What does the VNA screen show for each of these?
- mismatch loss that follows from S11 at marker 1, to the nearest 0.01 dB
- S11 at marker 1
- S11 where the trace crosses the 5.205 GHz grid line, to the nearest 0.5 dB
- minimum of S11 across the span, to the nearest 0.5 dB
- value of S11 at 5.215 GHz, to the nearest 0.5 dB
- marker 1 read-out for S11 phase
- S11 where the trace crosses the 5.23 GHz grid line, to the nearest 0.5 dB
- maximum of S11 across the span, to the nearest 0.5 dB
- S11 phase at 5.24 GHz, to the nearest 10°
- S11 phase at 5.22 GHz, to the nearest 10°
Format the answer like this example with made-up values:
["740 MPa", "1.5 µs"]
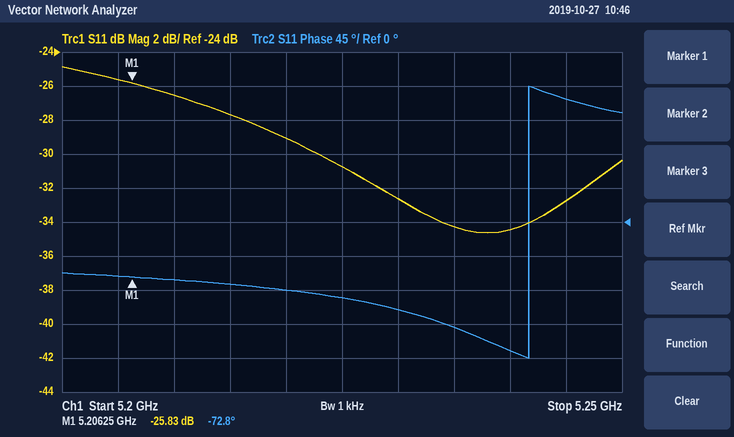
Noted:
["0.01 dB", "-25.83 dB", "-25.5 dB", "-34.5 dB", "-27.5 dB", "-72.8°", "-32.5 dB", "-25.0 dB", "-170°", "-90°"]
